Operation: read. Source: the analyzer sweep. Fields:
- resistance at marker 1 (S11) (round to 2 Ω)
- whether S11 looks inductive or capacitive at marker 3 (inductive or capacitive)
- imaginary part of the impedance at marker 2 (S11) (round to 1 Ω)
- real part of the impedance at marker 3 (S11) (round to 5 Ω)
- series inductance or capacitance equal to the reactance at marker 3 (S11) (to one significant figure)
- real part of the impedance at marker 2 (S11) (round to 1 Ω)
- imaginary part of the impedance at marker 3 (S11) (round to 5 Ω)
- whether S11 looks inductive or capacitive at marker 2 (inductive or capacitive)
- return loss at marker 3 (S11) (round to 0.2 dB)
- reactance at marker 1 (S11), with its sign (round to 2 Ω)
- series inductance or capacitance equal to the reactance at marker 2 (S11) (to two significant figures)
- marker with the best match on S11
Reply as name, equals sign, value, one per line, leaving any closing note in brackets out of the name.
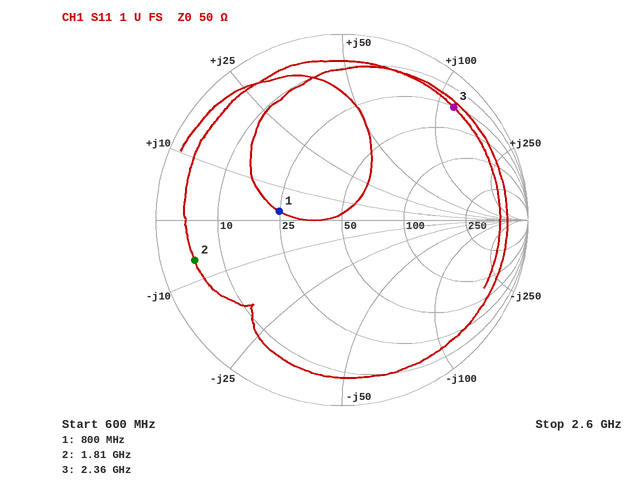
resistance at marker 1 (S11) = 24 Ω
whether S11 looks inductive or capacitive at marker 3 = inductive
imaginary part of the impedance at marker 2 (S11) = -7 Ω
real part of the impedance at marker 3 (S11) = 25 Ω
series inductance or capacitance equal to the reactance at marker 3 (S11) = 8 nH
real part of the impedance at marker 2 (S11) = 5 Ω
imaginary part of the impedance at marker 3 (S11) = +115 Ω
whether S11 looks inductive or capacitive at marker 2 = capacitive
return loss at marker 3 (S11) = 1.4 dB
reactance at marker 1 (S11), with its sign = +2 Ω
series inductance or capacitance equal to the reactance at marker 2 (S11) = 13 pF
marker with the best match on S11 = marker 1
